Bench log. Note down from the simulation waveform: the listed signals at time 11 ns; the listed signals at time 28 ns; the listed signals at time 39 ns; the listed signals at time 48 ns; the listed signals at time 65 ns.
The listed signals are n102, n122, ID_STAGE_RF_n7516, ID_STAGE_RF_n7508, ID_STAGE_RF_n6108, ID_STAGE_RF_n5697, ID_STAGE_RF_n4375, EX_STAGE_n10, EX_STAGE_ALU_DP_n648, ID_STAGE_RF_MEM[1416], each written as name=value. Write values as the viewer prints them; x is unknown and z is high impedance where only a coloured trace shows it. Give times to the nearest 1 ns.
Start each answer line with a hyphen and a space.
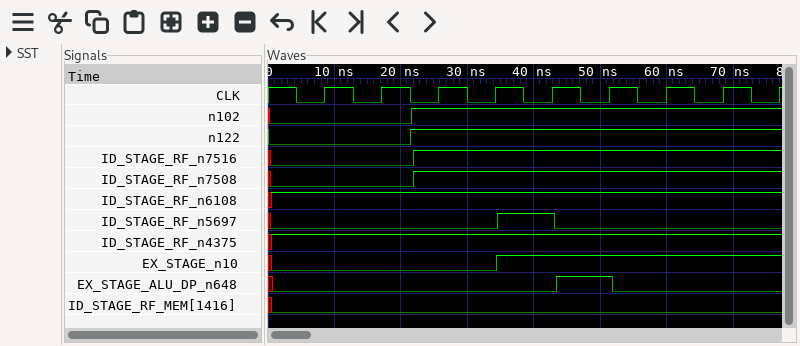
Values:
- n102=0, n122=0, ID_STAGE_RF_n7516=0, ID_STAGE_RF_n7508=0, ID_STAGE_RF_n6108=1, ID_STAGE_RF_n5697=0, ID_STAGE_RF_n4375=1, EX_STAGE_n10=0, EX_STAGE_ALU_DP_n648=0, ID_STAGE_RF_MEM[1416]=0
- n102=1, n122=1, ID_STAGE_RF_n7516=1, ID_STAGE_RF_n7508=1, ID_STAGE_RF_n6108=1, ID_STAGE_RF_n5697=0, ID_STAGE_RF_n4375=1, EX_STAGE_n10=0, EX_STAGE_ALU_DP_n648=0, ID_STAGE_RF_MEM[1416]=0
- n102=1, n122=1, ID_STAGE_RF_n7516=1, ID_STAGE_RF_n7508=1, ID_STAGE_RF_n6108=1, ID_STAGE_RF_n5697=1, ID_STAGE_RF_n4375=1, EX_STAGE_n10=1, EX_STAGE_ALU_DP_n648=0, ID_STAGE_RF_MEM[1416]=0
- n102=1, n122=1, ID_STAGE_RF_n7516=1, ID_STAGE_RF_n7508=1, ID_STAGE_RF_n6108=1, ID_STAGE_RF_n5697=0, ID_STAGE_RF_n4375=1, EX_STAGE_n10=1, EX_STAGE_ALU_DP_n648=1, ID_STAGE_RF_MEM[1416]=0
- n102=1, n122=1, ID_STAGE_RF_n7516=1, ID_STAGE_RF_n7508=1, ID_STAGE_RF_n6108=1, ID_STAGE_RF_n5697=0, ID_STAGE_RF_n4375=1, EX_STAGE_n10=1, EX_STAGE_ALU_DP_n648=0, ID_STAGE_RF_MEM[1416]=0
